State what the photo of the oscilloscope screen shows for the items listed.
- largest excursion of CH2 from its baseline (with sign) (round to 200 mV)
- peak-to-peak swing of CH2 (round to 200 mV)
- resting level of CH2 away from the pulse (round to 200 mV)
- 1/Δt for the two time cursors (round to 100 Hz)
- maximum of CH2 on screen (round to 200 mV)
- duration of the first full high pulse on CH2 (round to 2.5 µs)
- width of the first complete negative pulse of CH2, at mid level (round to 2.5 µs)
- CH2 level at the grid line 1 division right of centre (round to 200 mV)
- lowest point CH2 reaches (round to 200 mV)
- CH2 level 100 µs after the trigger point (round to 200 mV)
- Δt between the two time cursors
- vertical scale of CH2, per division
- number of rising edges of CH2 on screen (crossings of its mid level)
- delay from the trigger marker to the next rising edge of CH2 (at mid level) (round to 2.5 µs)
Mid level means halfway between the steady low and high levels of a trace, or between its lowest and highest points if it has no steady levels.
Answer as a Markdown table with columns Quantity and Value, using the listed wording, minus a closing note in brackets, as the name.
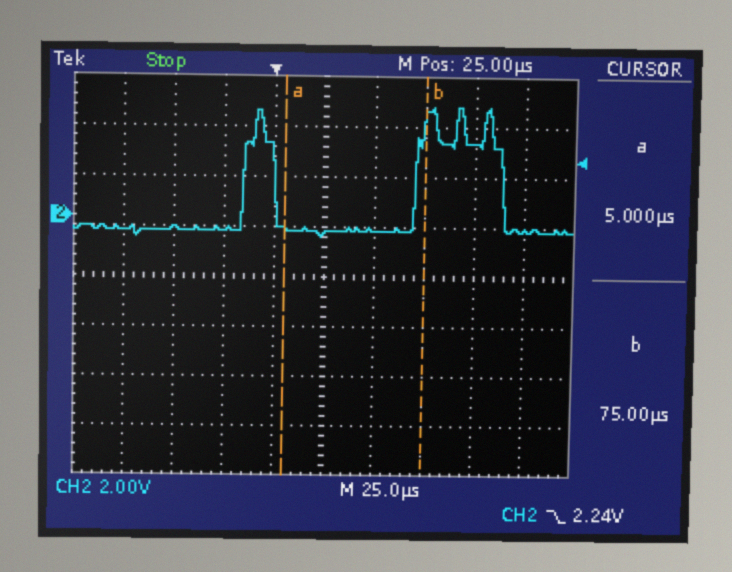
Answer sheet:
| Quantity | Value |
|---|---|
| largest excursion of CH2 from its baseline (with sign) | +5.0 V |
| peak-to-peak swing of CH2 | 5.2 V |
| resting level of CH2 away from the pulse | -600 mV |
| 1/Δt for the two time cursors | 14.3 kHz |
| maximum of CH2 on screen | 4.4 V |
| duration of the first full high pulse on CH2 | 15.0 µs |
| width of the first complete negative pulse of CH2, at mid level | 70.0 µs |
| CH2 level at the grid line 1 division right of centre | -600 mV |
| lowest point CH2 reaches | -800 mV |
| CH2 level 100 µs after the trigger point | 3.0 V |
| Δt between the two time cursors | 70.0 µs |
| vertical scale of CH2, per division | 2 V |
| number of rising edges of CH2 on screen | 2 |
| delay from the trigger marker to the next rising edge of CH2 (at mid level) | 70.0 µs |
